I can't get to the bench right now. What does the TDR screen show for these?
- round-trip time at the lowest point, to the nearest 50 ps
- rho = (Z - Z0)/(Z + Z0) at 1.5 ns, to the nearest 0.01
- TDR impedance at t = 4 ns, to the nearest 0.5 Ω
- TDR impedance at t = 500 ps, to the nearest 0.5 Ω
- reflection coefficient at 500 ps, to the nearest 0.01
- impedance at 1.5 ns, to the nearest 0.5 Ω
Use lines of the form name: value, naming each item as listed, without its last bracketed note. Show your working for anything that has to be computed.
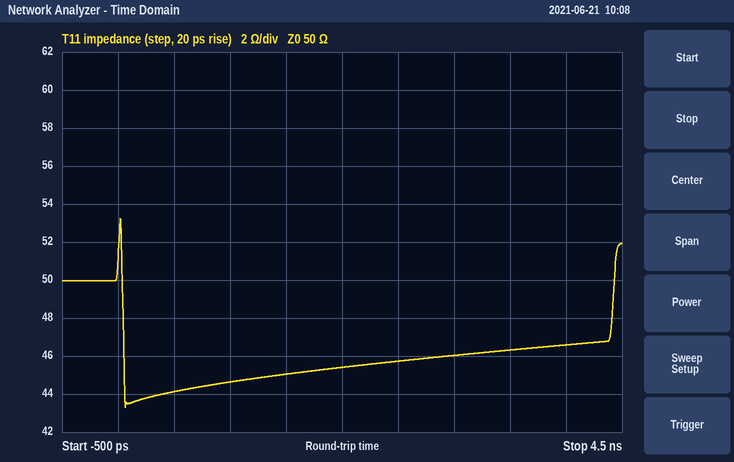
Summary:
round-trip time at the lowest point, to the nearest 50 ps: 50 ps
rho = (Z - Z0)/(Z + Z0) at 1.5 ns, to the nearest 0.01: (45 − 50)/(45 + 50) ≈ -0.05
TDR impedance at t = 4 ns, to the nearest 0.5 Ω: 46.5 Ω
TDR impedance at t = 500 ps, to the nearest 0.5 Ω: 44.0 Ω
reflection coefficient at 500 ps, to the nearest 0.01: (44 − 50)/(44 + 50) ≈ -0.06
impedance at 1.5 ns, to the nearest 0.5 Ω: 45.0 Ω
